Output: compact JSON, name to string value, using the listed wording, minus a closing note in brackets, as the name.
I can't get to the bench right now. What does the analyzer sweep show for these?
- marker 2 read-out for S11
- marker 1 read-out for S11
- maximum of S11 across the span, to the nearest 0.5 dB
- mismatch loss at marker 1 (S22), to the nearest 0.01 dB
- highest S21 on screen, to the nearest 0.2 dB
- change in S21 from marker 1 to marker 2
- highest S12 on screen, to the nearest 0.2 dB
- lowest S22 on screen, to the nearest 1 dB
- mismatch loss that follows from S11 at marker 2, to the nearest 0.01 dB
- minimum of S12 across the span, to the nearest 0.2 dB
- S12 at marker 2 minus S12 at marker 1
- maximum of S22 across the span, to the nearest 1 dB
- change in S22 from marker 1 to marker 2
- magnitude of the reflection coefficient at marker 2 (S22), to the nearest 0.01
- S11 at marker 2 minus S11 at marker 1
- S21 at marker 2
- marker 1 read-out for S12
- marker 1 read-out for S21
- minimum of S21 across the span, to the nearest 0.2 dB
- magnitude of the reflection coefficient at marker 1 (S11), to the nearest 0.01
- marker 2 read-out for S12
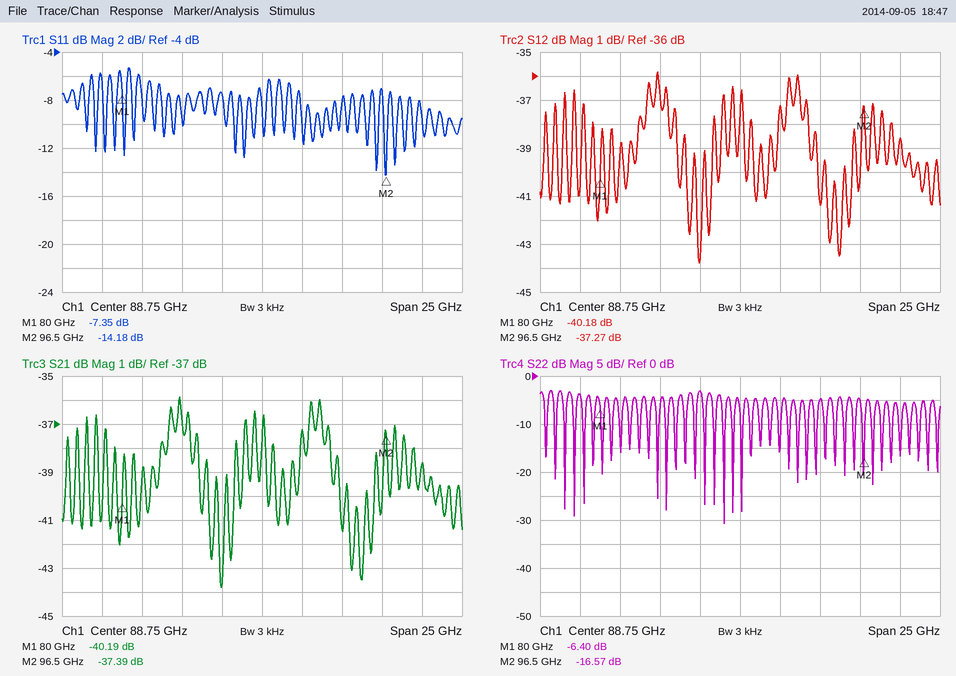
{"marker 2 read-out for S11": "-14.18 dB", "marker 1 read-out for S11": "-7.35 dB", "maximum of S11 across the span, to the nearest 0.5 dB": "-5.5 dB", "mismatch loss at marker 1 (S22), to the nearest 0.01 dB": "1.13 dB", "highest S21 on screen, to the nearest 0.2 dB": "-35.8 dB", "change in S21 from marker 1 to marker 2": "2.80 dB", "highest S12 on screen, to the nearest 0.2 dB": "-35.8 dB", "lowest S22 on screen, to the nearest 1 dB": "-31 dB", "mismatch loss that follows from S11 at marker 2, to the nearest 0.01 dB": "0.17 dB", "minimum of S12 across the span, to the nearest 0.2 dB": "-43.8 dB", "S12 at marker 2 minus S12 at marker 1": "2.91 dB", "maximum of S22 across the span, to the nearest 1 dB": "-3 dB", "change in S22 from marker 1 to marker 2": "-10.17 dB", "magnitude of the reflection coefficient at marker 2 (S22), to the nearest 0.01": "0.15", "S11 at marker 2 minus S11 at marker 1": "-6.83 dB", "S21 at marker 2": "-37.39 dB", "marker 1 read-out for S12": "-40.18 dB", "marker 1 read-out for S21": "-40.19 dB", "minimum of S21 across the span, to the nearest 0.2 dB": "-43.8 dB", "magnitude of the reflection coefficient at marker 1 (S11), to the nearest 0.01": "0.43", "marker 2 read-out for S12": "-37.27 dB"}
